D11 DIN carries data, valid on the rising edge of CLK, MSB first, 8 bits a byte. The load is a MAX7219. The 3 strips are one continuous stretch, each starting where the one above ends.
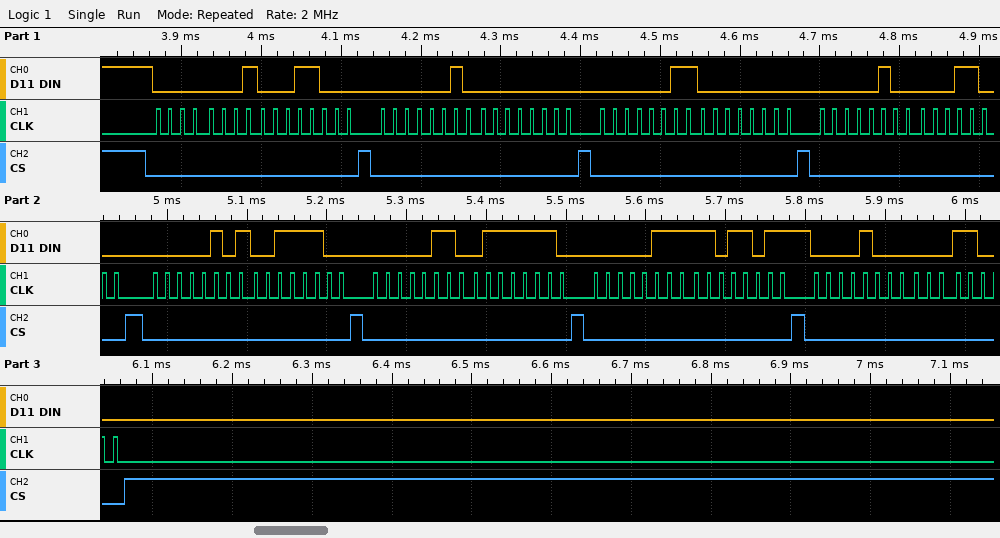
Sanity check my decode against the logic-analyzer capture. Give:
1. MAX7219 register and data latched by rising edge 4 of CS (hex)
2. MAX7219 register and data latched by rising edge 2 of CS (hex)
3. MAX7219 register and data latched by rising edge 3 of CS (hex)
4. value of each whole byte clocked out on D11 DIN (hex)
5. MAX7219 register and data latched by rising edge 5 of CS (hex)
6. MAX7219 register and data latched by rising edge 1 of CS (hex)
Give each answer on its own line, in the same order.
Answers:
register 0x4, data 0x18
register 0x2, data 0x00
register 0x3, data 0x00
01 18 02 00 03 00 04 18 05 3C 06 7E 07 DB 08 18
register 0x5, data 0x3C
register 0x1, data 0x18
